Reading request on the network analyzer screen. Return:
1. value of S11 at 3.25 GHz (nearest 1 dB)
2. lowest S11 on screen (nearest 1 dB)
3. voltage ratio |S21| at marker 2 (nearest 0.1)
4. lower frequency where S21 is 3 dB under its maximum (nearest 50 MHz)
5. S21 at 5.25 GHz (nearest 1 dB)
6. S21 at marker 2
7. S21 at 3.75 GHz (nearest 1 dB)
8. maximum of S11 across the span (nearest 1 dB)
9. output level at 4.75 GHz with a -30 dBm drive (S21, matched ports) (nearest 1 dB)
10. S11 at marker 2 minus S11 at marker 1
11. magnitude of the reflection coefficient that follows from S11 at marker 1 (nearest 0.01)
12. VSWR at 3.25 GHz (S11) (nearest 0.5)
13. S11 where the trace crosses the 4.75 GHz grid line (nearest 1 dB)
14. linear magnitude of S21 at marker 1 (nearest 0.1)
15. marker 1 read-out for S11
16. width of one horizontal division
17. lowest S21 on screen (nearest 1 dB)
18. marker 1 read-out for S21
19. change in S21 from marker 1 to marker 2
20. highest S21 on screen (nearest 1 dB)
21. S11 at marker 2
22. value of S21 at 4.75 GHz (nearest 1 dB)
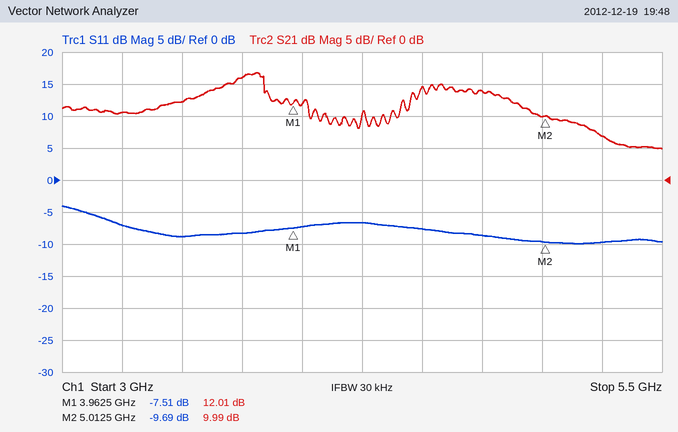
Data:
-7 dB
-10 dB
3.2
3.60 GHz
7 dB
9.99 dB
16 dB
-4 dB
-16 dBm
-2.18 dB
0.42
2.5
-9 dB
4.0
-7.51 dB
250 MHz
5 dB
12.01 dB
-2.02 dB
17 dB
-9.69 dB
14 dB
